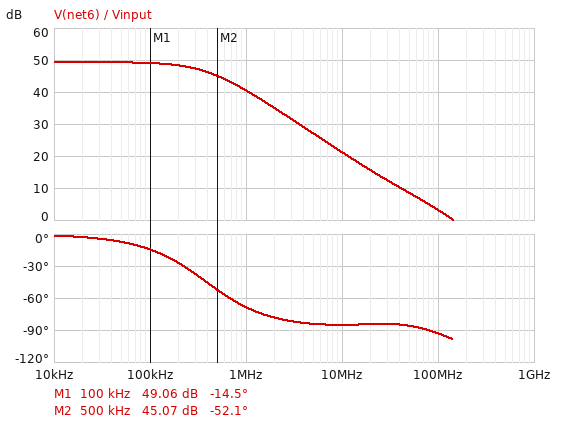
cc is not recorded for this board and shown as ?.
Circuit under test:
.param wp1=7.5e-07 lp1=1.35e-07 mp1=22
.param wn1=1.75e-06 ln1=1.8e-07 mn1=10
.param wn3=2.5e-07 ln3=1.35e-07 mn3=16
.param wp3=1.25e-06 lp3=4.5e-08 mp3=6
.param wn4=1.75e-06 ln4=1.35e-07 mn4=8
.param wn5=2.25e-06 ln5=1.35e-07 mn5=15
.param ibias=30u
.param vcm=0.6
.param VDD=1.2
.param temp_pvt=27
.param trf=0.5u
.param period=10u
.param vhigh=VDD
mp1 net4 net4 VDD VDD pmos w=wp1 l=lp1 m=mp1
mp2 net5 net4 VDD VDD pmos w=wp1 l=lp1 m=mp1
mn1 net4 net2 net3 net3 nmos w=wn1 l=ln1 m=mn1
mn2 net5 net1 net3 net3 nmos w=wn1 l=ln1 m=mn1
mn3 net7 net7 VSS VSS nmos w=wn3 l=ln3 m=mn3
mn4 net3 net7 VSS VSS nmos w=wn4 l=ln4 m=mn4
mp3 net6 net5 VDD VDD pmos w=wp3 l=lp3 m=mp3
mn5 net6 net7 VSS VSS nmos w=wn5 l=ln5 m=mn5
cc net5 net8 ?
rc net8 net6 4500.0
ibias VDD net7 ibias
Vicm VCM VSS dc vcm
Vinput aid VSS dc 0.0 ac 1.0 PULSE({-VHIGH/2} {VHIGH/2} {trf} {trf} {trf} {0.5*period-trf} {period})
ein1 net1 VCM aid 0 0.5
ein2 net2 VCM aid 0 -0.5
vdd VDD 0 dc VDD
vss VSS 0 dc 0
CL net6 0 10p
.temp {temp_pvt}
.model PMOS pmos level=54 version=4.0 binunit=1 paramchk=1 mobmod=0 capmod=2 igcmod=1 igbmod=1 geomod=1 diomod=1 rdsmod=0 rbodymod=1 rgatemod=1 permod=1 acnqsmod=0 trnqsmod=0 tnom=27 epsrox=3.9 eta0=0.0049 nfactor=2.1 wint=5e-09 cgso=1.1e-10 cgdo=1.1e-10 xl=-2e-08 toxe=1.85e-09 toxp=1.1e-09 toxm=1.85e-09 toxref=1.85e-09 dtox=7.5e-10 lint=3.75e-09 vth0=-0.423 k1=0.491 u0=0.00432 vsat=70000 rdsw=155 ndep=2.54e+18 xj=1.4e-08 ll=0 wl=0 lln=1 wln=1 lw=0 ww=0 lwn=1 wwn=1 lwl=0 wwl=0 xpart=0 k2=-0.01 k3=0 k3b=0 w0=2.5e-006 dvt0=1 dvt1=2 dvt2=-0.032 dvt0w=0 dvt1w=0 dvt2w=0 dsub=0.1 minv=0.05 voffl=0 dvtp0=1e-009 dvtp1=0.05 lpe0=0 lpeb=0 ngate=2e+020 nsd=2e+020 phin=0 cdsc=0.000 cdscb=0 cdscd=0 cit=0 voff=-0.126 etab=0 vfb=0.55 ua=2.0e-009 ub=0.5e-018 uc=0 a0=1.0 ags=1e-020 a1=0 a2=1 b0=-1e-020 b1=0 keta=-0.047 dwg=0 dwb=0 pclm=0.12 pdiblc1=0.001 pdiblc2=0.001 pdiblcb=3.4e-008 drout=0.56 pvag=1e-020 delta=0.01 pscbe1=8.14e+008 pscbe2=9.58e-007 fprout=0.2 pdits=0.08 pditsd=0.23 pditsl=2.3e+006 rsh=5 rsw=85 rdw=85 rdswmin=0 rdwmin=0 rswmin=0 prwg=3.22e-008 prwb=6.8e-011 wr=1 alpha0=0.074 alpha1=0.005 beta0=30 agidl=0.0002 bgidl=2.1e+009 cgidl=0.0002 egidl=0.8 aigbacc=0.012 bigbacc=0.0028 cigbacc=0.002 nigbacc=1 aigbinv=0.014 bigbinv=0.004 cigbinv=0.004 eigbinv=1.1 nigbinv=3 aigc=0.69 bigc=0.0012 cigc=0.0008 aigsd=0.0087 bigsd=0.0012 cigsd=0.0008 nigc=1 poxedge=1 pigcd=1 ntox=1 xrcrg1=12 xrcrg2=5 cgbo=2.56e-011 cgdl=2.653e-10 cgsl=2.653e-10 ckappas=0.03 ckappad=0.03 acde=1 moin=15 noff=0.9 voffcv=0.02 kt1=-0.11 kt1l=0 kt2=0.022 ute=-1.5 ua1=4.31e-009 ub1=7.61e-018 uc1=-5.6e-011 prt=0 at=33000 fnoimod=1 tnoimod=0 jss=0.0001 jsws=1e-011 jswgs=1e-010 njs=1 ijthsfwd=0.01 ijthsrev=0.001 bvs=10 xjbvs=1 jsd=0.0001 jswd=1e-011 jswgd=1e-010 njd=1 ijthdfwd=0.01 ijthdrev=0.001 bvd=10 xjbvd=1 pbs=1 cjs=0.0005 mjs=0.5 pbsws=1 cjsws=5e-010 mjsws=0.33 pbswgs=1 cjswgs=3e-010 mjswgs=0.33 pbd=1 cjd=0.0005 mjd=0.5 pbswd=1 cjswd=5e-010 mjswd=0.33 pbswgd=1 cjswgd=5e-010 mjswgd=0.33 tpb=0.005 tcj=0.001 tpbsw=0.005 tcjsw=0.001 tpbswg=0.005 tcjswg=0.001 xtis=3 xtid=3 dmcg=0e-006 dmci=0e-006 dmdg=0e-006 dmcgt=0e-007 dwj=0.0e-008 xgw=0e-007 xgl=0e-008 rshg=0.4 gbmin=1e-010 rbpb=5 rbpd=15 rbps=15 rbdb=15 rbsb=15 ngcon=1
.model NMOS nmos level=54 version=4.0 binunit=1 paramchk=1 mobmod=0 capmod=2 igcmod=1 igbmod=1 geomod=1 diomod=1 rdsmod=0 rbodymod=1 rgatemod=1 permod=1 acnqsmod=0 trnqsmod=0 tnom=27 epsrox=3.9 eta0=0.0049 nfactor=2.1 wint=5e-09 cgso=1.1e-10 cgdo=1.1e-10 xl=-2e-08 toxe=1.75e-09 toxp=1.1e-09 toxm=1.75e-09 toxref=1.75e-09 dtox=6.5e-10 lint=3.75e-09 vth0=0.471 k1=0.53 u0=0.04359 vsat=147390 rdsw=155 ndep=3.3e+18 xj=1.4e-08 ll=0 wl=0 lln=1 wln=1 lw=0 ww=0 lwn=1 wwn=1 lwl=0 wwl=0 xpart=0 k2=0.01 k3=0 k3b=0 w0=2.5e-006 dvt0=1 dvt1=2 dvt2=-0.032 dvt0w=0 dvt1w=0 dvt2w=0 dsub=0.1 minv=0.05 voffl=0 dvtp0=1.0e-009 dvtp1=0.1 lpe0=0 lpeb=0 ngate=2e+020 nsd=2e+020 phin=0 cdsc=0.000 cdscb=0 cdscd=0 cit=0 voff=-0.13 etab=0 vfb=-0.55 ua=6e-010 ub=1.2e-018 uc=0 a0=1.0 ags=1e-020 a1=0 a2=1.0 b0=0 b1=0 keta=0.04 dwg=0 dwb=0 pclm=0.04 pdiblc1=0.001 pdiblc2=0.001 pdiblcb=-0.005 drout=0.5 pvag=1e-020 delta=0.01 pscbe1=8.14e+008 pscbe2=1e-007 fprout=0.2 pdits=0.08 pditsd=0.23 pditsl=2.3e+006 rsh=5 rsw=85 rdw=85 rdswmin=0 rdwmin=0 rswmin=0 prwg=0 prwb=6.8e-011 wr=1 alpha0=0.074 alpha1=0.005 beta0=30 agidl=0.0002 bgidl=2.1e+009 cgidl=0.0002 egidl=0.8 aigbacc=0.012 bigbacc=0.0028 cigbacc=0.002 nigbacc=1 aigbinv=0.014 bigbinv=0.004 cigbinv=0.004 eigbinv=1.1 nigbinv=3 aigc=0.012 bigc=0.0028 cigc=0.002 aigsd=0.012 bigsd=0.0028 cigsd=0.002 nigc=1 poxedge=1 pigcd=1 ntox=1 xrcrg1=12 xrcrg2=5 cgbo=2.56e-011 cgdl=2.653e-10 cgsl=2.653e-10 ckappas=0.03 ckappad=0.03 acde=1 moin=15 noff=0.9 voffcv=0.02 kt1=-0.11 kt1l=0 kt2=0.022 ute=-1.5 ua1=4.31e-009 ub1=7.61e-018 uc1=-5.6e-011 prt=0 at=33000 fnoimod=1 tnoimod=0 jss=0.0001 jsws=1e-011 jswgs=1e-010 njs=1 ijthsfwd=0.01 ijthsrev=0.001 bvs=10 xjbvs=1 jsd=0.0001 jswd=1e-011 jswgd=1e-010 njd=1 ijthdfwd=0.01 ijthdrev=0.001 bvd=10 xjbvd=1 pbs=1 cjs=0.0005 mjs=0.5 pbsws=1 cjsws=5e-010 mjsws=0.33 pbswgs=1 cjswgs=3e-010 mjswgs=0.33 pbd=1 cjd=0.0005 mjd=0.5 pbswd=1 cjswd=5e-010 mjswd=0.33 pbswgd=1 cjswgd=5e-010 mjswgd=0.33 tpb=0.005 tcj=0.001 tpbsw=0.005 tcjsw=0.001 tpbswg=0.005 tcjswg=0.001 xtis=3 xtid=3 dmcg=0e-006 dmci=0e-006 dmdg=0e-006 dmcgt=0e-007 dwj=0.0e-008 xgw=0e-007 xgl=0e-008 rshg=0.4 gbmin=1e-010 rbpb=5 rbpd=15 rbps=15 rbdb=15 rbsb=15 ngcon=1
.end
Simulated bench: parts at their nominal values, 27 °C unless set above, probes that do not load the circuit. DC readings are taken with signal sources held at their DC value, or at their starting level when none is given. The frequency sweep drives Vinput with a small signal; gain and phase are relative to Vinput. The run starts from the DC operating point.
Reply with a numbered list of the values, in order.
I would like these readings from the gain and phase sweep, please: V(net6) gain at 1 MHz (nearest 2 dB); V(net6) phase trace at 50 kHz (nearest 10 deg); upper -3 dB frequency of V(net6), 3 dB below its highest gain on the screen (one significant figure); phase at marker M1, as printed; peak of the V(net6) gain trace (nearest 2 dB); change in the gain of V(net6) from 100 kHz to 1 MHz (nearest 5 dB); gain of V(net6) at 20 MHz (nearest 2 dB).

1. 40 dB
2. -10 deg
3. 400 kHz
4. -14.5 deg
5. 50 dB
6. -10 dB
7. 16 dB
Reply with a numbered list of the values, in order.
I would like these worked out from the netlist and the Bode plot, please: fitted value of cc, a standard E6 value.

1. 1 pF
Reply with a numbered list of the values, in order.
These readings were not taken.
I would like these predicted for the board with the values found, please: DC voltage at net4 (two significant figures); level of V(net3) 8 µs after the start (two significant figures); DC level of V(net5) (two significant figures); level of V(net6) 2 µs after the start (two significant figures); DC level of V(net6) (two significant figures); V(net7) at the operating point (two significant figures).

1. 670 mV
2. 420 mV
3. 670 mV
4. 1.2 V
5. 930 mV
6. 470 mV
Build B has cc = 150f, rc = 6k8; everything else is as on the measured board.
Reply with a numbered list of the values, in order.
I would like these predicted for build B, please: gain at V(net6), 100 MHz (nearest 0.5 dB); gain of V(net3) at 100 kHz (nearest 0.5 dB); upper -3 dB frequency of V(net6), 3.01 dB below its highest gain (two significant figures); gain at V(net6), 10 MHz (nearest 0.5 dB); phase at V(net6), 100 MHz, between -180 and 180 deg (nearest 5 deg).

1. 10.5 dB
2. -13.0 dB
3. 2.1 MHz
4. 35.5 dB
5. -130 deg
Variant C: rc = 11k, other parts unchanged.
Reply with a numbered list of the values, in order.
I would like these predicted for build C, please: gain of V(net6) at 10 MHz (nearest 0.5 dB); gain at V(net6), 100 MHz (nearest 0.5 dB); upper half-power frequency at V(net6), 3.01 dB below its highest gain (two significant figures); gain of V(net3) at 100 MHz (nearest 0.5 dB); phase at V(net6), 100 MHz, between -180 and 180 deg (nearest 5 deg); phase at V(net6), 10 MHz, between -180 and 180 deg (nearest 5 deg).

1. 22.5 dB
2. 10.5 dB
3. 380 kHz
4. -25.0 dB
5. -90 deg
6. -65 deg
